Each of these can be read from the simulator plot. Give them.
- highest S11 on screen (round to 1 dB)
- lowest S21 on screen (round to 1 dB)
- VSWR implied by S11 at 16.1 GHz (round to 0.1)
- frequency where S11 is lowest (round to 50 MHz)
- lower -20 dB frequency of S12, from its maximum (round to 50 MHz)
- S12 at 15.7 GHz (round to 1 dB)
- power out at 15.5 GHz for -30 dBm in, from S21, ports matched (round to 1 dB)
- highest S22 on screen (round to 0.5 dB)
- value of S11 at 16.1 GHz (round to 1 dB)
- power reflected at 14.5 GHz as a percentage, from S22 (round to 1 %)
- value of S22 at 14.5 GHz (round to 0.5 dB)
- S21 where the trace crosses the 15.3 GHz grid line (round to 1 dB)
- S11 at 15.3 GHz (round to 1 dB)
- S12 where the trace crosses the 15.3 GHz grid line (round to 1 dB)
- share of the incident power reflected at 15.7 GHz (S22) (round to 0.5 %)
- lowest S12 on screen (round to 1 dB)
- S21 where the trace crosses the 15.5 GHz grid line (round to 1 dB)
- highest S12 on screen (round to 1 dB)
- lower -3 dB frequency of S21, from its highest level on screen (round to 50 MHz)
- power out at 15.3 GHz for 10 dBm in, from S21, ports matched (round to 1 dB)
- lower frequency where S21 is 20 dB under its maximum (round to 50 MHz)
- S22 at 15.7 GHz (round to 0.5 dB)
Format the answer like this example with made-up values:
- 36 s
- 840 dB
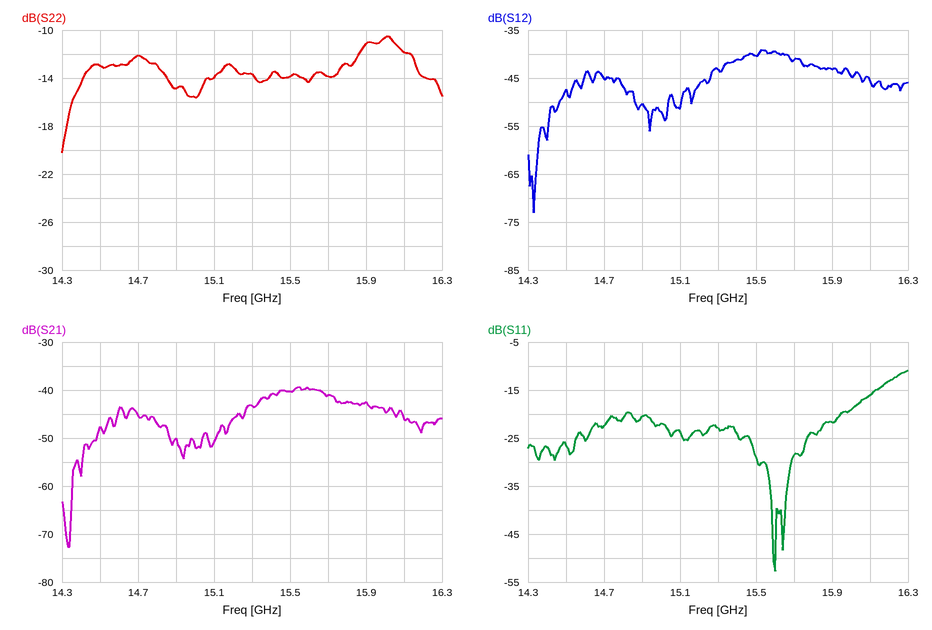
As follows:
- -11 dB
- -73 dB
- 1.4
- 15.60 GHz
- 14.35 GHz
- -41 dB
- -70 dBm
- -10.5 dB
- -16 dB
- 5 %
- -13.0 dB
- -43 dB
- -23 dB
- -43 dB
- 4.0 %
- -73 dB
- -40 dB
- -39 dB
- 15.35 GHz
- -33 dBm
- 14.35 GHz
- -14.0 dB
